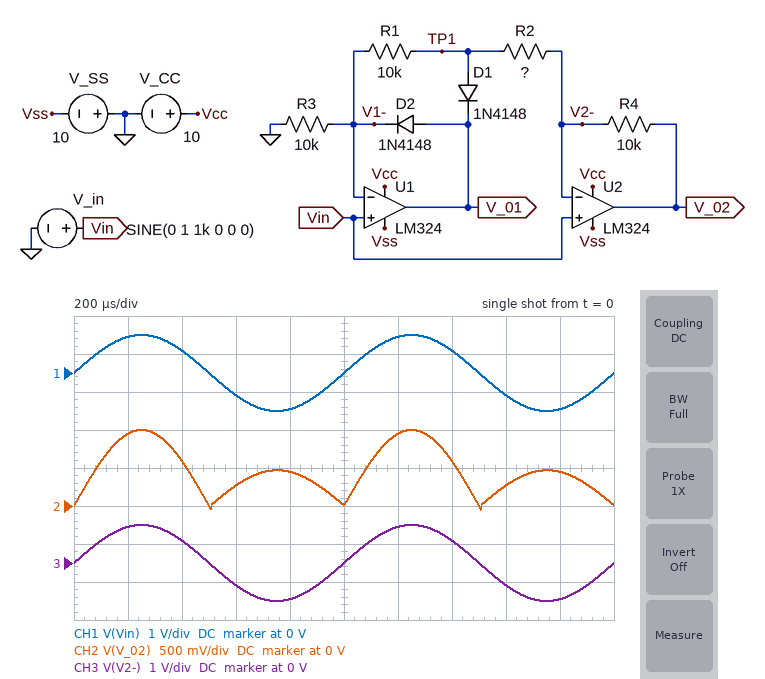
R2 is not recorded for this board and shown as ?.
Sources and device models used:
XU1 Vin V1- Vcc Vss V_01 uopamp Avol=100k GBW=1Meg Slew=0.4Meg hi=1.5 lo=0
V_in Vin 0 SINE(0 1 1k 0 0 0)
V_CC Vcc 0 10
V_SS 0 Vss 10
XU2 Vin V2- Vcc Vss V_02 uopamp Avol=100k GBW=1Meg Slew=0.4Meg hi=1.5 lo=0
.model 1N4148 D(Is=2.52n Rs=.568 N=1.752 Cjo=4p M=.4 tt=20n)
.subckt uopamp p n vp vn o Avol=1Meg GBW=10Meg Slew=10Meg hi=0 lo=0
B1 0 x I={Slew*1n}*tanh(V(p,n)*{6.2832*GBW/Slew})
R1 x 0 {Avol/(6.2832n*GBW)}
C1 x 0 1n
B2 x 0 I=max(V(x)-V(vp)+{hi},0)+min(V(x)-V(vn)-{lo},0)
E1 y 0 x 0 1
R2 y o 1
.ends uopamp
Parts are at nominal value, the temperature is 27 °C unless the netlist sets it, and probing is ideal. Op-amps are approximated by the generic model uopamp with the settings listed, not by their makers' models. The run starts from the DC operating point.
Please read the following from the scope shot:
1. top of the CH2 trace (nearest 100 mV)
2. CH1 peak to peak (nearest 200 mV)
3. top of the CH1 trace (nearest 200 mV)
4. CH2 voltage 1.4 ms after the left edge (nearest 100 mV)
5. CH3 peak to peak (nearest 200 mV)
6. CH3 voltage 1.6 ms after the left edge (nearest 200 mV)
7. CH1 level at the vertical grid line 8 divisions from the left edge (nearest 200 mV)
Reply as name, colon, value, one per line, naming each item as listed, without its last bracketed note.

top of the CH2 trace: 1.0 V
CH1 peak to peak: 2.0 V
top of the CH1 trace: 1.0 V
CH2 voltage 1.4 ms after the left edge: 600 mV
CH3 peak to peak: 2.0 V
CH3 voltage 1.6 ms after the left edge: -600 mV
CH1 level at the vertical grid line 8 divisions from the left edge: -600 mV
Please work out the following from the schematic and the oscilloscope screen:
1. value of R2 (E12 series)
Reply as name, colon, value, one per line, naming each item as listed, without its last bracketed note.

value of R2: 6.8 kΩ
